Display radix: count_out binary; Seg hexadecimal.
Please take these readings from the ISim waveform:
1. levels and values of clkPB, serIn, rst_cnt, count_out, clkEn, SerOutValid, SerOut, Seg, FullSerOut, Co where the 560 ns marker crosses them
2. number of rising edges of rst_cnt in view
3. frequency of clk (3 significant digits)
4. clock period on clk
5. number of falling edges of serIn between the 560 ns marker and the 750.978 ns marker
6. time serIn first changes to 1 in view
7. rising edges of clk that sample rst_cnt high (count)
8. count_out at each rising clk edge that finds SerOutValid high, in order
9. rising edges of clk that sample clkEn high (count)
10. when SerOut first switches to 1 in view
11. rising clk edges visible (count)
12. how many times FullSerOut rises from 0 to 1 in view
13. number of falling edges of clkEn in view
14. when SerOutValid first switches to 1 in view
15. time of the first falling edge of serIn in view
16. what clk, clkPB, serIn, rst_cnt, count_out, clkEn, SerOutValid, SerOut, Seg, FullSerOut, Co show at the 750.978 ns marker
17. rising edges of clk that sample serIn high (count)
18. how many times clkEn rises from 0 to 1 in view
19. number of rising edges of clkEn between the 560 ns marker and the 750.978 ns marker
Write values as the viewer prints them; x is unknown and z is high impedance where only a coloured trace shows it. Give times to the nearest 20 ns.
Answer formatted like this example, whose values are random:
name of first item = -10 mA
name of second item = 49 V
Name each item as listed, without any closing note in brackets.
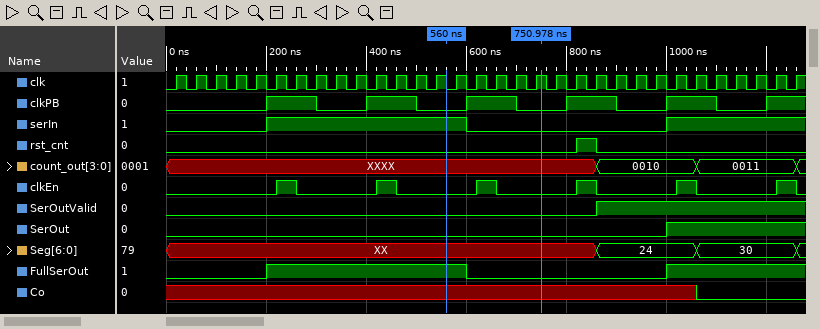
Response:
levels and values of clkPB, serIn, rst_cnt, count_out, clkEn, SerOutValid, SerOut, Seg, FullSerOut, Co where the 560 ns marker crosses them = clkPB=0, serIn=1, rst_cnt=0, count_out=XXXX, clkEn=0, SerOutValid=0, SerOut=0, Seg=XX, FullSerOut=1, Co=x
number of rising edges of rst_cnt in view = 1
frequency of clk = 25.0 MHz
clock period on clk = 40 ns
number of falling edges of serIn between the 560 ns marker and the 750.978 ns marker = 1
time serIn first changes to 1 in view = 200 ns
rising edges of clk that sample rst_cnt high = 1
count_out at each rising clk edge that finds SerOutValid high, in order = 0010, 0010, 0010, 0010, 0010, 0011, 0011, 0011, 0011, 0011
rising edges of clk that sample clkEn high = 6
when SerOut first switches to 1 in view = 1000 ns
rising clk edges visible = 32
how many times FullSerOut rises from 0 to 1 in view = 2
number of falling edges of clkEn in view = 6
when SerOutValid first switches to 1 in view = 860 ns
time of the first falling edge of serIn in view = 600 ns
what clk, clkPB, serIn, rst_cnt, count_out, clkEn, SerOutValid, SerOut, Seg, FullSerOut, Co show at the 750.978 ns marker = clk=1, clkPB=0, serIn=0, rst_cnt=0, count_out=XXXX, clkEn=0, SerOutValid=0, SerOut=0, Seg=XX, FullSerOut=0, Co=x
rising edges of clk that sample serIn high = 17
how many times clkEn rises from 0 to 1 in view = 6
number of rising edges of clkEn between the 560 ns marker and the 750.978 ns marker = 1
